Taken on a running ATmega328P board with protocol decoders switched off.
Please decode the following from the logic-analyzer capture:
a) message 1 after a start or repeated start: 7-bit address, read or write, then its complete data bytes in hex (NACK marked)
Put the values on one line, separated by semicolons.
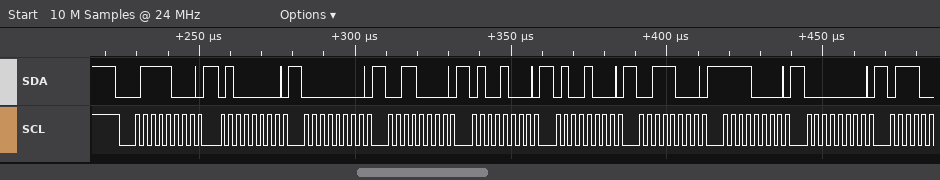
0x3C write: 40 00 30 48 48 38 F0 00
